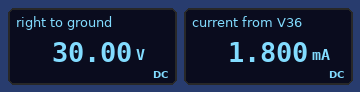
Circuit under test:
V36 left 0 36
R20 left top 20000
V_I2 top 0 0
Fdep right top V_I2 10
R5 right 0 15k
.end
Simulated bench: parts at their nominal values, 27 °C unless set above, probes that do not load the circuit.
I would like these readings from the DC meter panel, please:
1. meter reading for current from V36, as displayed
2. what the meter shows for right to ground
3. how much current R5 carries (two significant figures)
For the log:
1.800 mA
30.00 V
2.0 mA
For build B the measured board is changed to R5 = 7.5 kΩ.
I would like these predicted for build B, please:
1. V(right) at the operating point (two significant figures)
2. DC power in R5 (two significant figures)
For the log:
15 V
30 mW
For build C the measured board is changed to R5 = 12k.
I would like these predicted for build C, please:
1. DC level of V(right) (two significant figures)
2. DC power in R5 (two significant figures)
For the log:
24 V
48 mW
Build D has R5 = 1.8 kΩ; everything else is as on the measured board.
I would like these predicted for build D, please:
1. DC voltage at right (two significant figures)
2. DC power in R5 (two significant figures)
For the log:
3.6 V
7.2 mW
